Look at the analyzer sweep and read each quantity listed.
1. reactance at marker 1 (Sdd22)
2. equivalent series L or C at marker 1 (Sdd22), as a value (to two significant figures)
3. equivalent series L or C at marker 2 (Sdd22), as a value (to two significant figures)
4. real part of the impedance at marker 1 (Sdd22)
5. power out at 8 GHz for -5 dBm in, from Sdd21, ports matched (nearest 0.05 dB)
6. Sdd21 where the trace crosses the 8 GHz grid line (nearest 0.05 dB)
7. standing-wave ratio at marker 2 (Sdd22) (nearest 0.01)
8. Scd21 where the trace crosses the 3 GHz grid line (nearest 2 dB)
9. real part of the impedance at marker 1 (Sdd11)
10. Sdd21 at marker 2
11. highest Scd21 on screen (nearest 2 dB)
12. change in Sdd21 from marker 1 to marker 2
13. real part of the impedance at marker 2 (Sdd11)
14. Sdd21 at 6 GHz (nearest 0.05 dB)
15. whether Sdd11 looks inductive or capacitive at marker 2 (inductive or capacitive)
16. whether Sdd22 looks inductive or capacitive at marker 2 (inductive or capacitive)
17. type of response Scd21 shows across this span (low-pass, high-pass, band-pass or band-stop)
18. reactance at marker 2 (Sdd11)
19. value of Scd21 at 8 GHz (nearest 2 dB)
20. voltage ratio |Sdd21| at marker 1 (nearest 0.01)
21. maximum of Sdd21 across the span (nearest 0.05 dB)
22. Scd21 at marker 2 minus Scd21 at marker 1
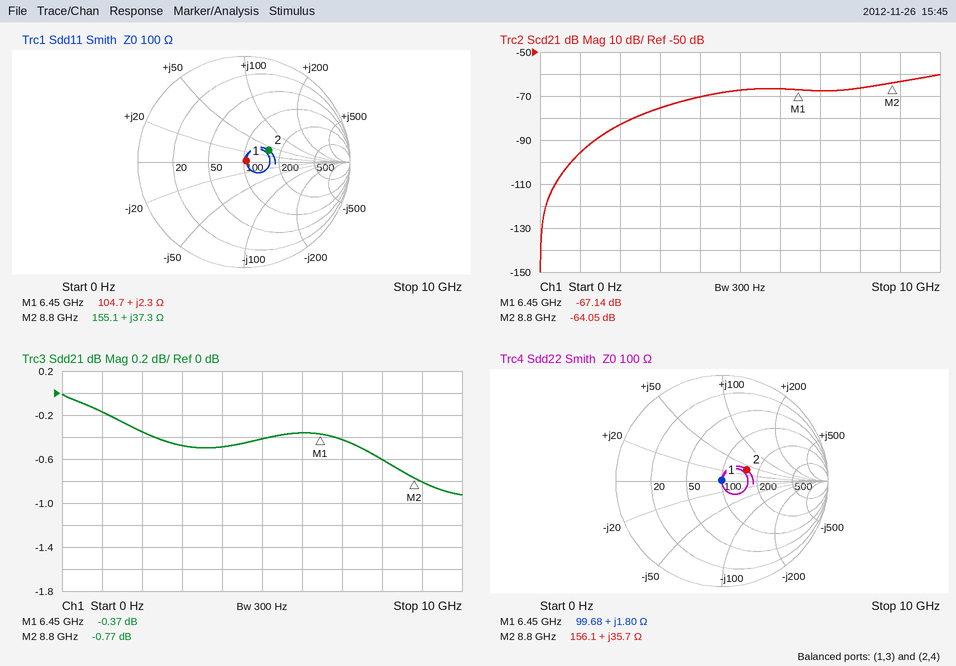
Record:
+1.80 Ω
44 pH
650 pH
99.68 Ω
-5.60 dBm
-0.60 dB
1.69
-76 dB
104.7 Ω
-0.77 dB
-60 dB
-0.40 dB
155.1 Ω
-0.35 dB
inductive
inductive
high-pass
+37.3 Ω
-66 dB
0.96
0.00 dB
3.09 dB
